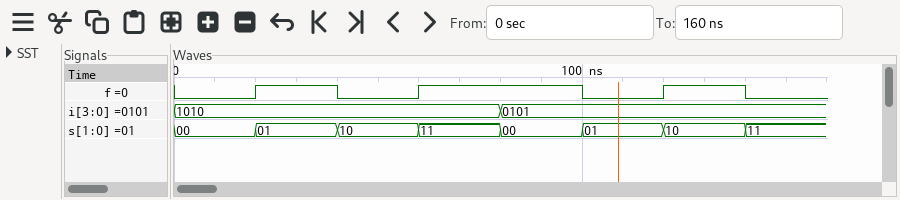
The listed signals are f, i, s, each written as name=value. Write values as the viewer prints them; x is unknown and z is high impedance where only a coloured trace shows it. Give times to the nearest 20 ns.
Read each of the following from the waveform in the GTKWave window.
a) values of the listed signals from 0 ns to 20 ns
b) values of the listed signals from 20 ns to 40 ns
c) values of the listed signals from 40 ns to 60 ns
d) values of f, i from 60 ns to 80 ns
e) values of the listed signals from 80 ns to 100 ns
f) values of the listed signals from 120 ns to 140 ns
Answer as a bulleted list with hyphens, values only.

- f=0, i=1010, s=00
- f=1, i=1010, s=01
- f=0, i=1010, s=10
- f=1, i=1010
- f=1, i=0101, s=00
- f=1, i=0101, s=10
